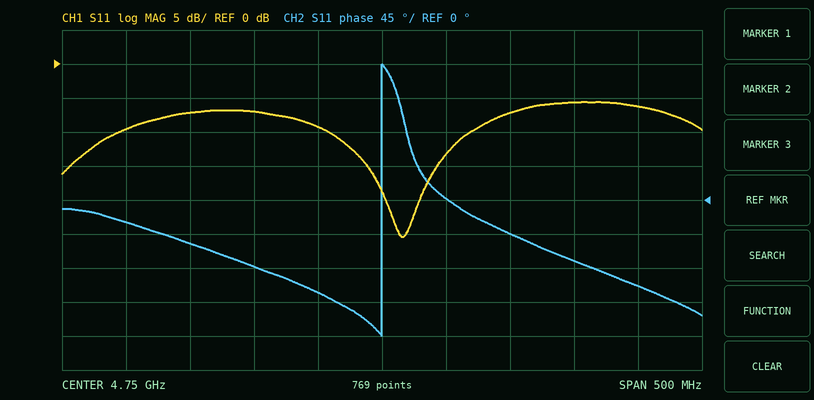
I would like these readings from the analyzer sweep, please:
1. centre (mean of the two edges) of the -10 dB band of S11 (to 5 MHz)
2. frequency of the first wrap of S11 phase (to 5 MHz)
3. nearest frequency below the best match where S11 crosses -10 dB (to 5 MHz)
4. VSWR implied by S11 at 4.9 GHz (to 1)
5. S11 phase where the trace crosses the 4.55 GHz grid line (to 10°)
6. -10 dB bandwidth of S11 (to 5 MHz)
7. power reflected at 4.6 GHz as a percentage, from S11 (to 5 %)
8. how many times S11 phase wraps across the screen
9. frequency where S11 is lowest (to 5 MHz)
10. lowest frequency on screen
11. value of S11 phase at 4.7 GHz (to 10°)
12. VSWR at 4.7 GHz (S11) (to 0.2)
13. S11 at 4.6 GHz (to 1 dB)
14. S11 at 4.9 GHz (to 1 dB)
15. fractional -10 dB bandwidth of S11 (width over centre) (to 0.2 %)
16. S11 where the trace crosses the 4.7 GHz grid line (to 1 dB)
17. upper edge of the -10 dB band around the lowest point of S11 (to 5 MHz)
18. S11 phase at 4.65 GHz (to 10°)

4.765 GHz
4.750 GHz
4.710 GHz
3
-30°
110 MHz
20 %
1
4.765 GHz
4.5 GHz
-120°
2.0
-7 dB
-6 dB
2.4 %
-9 dB
4.820 GHz
-90°
